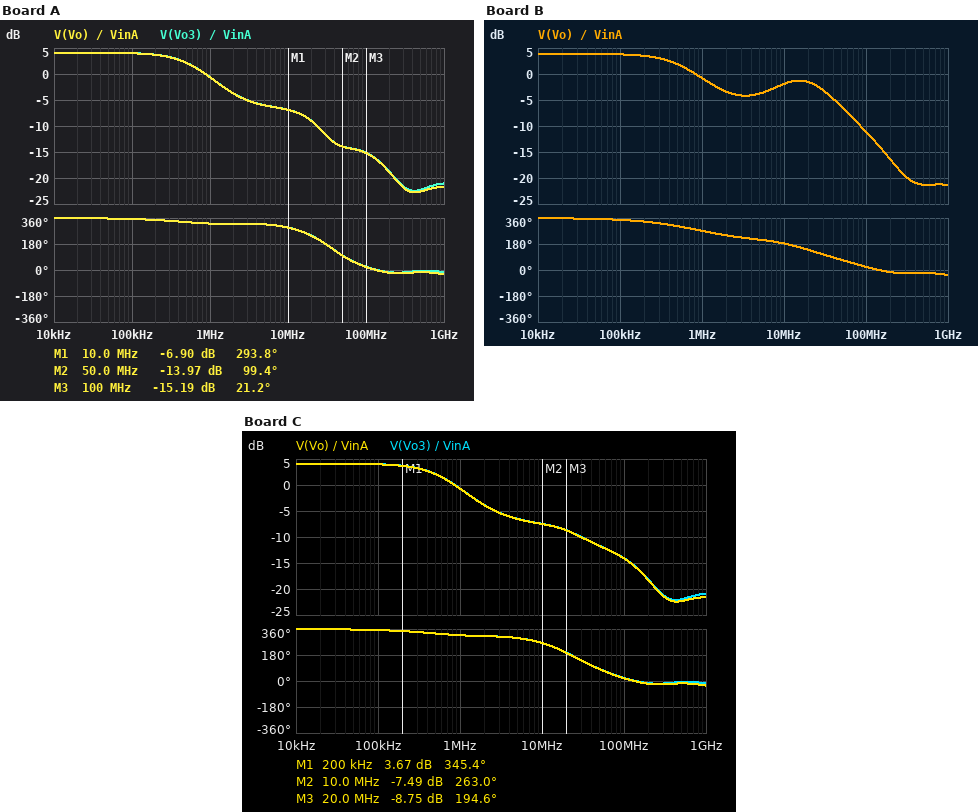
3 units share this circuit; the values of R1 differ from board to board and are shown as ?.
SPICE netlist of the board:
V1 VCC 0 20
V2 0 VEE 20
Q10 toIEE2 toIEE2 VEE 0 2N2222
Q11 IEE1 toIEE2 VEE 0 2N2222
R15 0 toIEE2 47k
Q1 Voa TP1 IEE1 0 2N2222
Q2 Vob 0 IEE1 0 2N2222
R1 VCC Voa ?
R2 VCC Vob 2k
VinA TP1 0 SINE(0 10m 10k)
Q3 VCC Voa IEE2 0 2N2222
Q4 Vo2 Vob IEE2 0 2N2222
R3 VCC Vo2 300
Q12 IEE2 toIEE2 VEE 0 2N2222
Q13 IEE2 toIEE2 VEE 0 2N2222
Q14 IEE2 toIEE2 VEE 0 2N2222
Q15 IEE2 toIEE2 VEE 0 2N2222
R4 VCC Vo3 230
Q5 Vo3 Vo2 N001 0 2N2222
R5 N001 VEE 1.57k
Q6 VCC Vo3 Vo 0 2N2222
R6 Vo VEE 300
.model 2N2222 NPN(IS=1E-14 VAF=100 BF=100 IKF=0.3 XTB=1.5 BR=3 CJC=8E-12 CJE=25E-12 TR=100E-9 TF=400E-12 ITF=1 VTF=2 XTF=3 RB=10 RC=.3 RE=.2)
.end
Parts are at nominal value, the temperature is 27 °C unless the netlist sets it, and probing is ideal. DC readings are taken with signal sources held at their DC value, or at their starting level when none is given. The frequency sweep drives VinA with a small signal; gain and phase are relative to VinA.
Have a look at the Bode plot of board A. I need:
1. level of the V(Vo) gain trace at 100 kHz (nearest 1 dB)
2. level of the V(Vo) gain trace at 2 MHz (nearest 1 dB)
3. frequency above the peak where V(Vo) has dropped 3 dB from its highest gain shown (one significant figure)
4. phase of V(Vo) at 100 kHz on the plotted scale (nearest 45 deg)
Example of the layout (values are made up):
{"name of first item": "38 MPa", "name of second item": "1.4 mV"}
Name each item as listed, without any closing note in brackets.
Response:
{"level of the V(Vo) gain trace at 100 kHz": "4 dB", "level of the V(Vo) gain trace at 2 MHz": "-4 dB", "frequency above the peak where V(Vo) has dropped 3 dB from its highest gain shown": "700 kHz", "phase of V(Vo) at 100 kHz on the plotted scale": "360 deg"}
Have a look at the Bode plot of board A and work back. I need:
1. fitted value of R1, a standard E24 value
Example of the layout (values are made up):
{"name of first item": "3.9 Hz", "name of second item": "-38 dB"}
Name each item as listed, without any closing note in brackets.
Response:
{"fitted value of R1, a standard E24 value": "750 Ω"}
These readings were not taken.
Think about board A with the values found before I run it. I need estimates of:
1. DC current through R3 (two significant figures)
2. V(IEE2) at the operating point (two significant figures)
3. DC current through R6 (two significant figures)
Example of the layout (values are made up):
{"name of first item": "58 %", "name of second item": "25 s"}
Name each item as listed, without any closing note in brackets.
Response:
{"DC current through R3": "8.1 mA", "V(IEE2) at the operating point": "19 V", "DC current through R6": "120 mA"}
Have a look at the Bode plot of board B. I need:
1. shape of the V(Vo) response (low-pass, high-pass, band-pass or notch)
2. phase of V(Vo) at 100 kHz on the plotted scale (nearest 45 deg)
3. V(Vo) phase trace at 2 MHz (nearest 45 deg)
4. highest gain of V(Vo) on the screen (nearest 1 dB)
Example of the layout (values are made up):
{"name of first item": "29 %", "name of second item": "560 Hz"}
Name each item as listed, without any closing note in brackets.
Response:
{"shape of the V(Vo) response": "low-pass", "phase of V(Vo) at 100 kHz on the plotted scale": "360 deg", "V(Vo) phase trace at 2 MHz": "225 deg", "highest gain of V(Vo) on the screen": "4 dB"}
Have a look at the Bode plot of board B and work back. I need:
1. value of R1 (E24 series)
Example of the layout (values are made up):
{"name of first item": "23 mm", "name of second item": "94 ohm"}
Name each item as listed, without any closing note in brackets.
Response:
{"value of R1": "5.6 kΩ"}
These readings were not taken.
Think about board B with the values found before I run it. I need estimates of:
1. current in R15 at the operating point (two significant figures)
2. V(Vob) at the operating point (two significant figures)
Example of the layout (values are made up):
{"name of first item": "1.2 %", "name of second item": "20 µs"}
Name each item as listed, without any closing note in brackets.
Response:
{"current in R15 at the operating point": "410 µA", "V(Vob) at the operating point": "18 V"}
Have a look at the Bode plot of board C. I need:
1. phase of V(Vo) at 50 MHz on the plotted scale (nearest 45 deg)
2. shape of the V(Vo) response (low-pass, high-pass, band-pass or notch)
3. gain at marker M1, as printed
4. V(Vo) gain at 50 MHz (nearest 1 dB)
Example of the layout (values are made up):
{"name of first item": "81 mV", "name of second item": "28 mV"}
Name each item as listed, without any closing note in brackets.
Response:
{"phase of V(Vo) at 50 MHz on the plotted scale": "90 deg", "shape of the V(Vo) response": "low-pass", "gain at marker M1, as printed": "3.67 dB", "V(Vo) gain at 50 MHz": "-12 dB"}
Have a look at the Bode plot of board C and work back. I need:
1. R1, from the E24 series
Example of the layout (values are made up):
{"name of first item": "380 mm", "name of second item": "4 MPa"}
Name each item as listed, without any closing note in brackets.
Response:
{"R1, from the E24 series": "1.5 kΩ"}
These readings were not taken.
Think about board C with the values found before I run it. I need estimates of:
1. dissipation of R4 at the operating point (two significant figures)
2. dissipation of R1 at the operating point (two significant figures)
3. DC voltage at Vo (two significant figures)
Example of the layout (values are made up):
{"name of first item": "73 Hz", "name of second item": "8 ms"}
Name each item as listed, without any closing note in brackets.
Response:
{"dissipation of R4 at the operating point": "47 mW", "dissipation of R1 at the operating point": "110 µW", "DC voltage at Vo": "16 V"}
